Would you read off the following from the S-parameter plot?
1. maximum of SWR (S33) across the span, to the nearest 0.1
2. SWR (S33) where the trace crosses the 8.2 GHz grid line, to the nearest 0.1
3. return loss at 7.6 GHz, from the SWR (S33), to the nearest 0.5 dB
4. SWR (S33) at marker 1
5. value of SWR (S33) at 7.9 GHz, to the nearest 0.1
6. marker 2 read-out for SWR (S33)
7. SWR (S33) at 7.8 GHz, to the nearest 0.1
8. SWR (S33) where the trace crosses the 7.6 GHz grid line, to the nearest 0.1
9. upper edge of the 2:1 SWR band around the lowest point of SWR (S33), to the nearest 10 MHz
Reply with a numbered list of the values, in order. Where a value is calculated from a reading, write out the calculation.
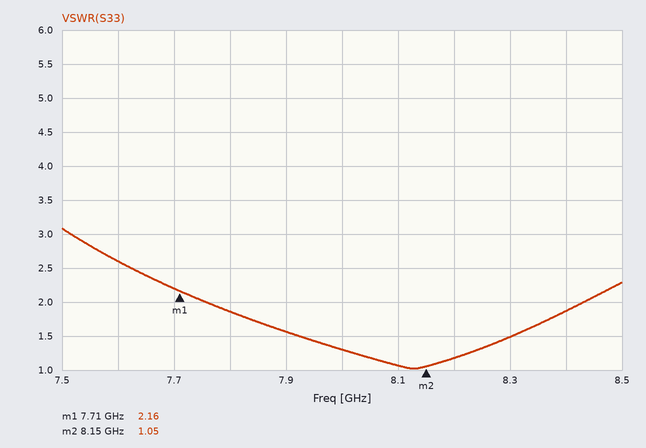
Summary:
1. 3.1
2. 1.2
3. −20 log10((2.6 − 1)/(2.6 + 1)) ≈ 7.0 dB
4. 2.16
5. 1.6
6. 1.05
7. 1.9
8. 2.6
9. 8.43 GHz
